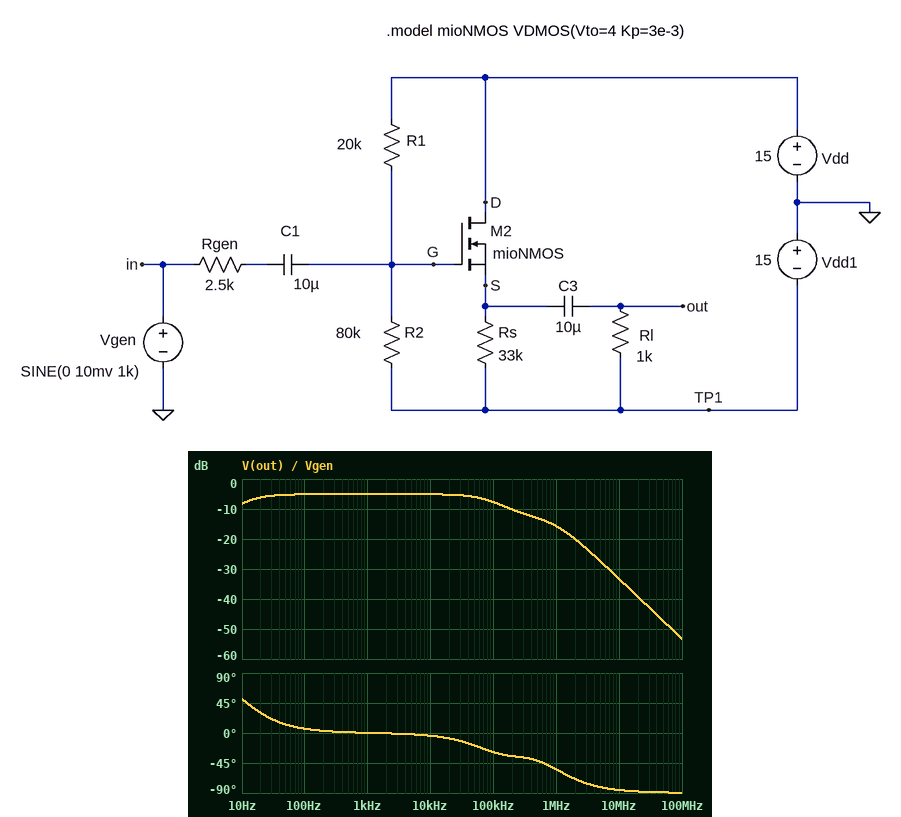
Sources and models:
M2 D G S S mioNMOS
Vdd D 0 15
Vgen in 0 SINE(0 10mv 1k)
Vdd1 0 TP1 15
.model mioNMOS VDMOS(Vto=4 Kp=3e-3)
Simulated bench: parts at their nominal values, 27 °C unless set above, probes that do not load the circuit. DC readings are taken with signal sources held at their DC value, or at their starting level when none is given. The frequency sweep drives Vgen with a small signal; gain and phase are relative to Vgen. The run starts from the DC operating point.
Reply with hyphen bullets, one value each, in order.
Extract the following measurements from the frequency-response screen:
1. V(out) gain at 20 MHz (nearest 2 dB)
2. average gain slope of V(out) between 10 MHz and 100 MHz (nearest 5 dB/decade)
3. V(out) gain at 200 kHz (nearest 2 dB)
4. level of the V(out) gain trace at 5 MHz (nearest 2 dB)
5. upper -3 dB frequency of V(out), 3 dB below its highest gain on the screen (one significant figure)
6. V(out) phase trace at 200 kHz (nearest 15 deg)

- -40 dB
- -20 dB/decade
- -10 dB
- -28 dB
- 100 kHz
- -30 deg
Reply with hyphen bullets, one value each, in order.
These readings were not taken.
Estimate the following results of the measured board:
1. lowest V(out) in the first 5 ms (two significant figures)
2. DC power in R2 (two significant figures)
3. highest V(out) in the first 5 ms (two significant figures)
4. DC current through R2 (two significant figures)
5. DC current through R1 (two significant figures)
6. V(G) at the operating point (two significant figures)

- -15 V
- 7.2 mW
- -15 V
- 300 µA
- 300 µA
- 9.0 V
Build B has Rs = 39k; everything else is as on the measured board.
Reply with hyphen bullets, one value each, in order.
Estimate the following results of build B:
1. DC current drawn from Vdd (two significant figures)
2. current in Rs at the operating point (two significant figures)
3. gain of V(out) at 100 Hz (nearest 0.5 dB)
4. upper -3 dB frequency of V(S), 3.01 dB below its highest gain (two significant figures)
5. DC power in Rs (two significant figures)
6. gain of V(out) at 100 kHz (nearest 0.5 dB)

- 800 µA
- 500 µA
- -5.5 dB
- 39 Hz
- 9.7 mW
- -8.0 dB
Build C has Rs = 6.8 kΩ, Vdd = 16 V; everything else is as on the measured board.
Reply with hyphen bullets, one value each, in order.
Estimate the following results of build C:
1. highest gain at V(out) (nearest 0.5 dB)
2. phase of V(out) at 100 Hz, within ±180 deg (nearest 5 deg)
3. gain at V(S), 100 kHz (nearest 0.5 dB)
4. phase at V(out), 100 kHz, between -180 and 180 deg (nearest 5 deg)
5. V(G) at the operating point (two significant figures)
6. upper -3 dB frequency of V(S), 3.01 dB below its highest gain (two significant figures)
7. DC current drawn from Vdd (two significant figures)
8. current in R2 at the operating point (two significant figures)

- -3.5 dB
- 10 deg
- -5.0 dB
- -30 deg
- 9.8 V
- 98 kHz
- 3.2 mA
- 310 µA
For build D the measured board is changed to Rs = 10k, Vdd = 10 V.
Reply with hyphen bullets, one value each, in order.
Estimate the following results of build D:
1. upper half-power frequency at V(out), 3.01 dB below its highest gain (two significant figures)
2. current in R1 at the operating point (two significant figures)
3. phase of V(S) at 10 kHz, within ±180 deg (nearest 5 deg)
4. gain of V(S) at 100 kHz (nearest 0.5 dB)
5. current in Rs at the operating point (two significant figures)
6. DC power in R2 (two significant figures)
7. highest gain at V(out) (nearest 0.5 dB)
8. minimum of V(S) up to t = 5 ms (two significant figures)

- 130 kHz
- 250 µA
- -5 deg
- -6.0 dB
- 1.5 mA
- 5.0 mW
- -4.0 dB
- -6.3 mV
